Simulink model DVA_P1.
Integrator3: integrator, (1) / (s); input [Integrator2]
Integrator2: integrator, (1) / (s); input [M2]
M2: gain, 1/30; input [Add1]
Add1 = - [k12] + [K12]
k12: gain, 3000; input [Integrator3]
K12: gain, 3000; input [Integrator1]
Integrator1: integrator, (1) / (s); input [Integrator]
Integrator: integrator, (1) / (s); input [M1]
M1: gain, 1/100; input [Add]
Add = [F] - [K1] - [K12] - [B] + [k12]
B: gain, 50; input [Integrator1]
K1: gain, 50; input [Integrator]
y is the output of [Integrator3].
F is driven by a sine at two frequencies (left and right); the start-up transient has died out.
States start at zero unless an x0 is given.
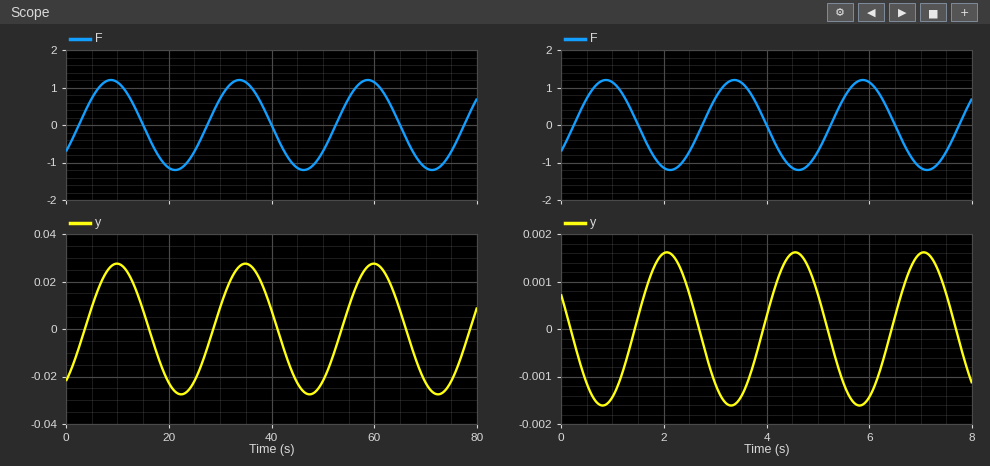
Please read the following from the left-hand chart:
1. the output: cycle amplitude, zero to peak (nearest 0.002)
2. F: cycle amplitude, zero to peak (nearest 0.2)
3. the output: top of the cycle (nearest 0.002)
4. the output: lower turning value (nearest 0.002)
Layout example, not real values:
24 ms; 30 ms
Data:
0.028; 1.2; 0.028; -0.028
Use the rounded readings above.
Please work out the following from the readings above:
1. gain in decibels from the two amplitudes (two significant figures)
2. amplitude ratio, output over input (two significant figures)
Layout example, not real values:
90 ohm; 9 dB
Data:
-33 dB; 0.023
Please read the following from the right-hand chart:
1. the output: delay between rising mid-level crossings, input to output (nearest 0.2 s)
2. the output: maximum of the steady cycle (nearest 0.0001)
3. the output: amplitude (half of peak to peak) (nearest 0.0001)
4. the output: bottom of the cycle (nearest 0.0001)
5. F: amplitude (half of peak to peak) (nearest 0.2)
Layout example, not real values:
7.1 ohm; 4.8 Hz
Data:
1.2 s; 0.0016; 0.0016; -0.0016; 1.2
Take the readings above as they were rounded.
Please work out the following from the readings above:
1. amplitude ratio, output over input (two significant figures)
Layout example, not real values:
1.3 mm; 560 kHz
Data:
0.0013
